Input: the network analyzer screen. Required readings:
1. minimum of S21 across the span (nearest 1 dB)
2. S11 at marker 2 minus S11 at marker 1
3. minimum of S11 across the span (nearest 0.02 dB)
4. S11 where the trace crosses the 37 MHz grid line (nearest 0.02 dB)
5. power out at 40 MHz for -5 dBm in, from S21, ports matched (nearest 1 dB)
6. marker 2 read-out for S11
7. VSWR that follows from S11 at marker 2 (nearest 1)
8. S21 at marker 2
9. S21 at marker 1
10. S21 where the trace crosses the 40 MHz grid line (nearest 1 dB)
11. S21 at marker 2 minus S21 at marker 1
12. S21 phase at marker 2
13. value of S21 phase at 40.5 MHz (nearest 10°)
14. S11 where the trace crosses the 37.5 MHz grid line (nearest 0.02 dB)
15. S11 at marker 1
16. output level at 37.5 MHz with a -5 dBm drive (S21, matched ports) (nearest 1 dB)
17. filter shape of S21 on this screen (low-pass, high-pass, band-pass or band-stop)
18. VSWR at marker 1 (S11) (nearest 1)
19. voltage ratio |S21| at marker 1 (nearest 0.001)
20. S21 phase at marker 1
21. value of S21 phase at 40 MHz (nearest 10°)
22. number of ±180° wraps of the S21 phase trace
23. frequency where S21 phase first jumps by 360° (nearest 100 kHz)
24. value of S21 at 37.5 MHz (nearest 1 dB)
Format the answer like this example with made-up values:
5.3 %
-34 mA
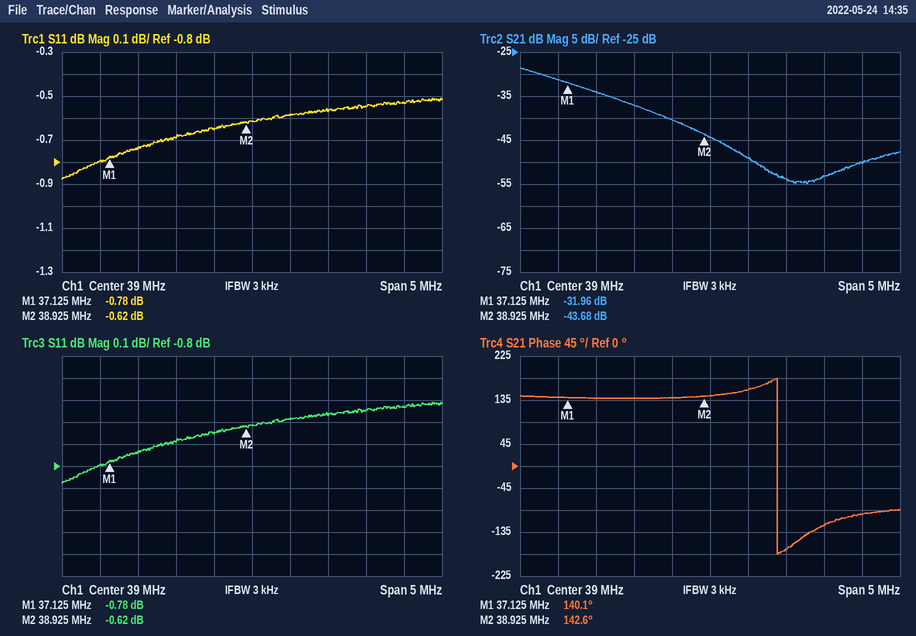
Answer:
-55 dB
0.16 dB
-0.88 dB
-0.80 dB
-59 dBm
-0.62 dB
28
-43.68 dB
-31.96 dB
-54 dB
-11.72 dB
142.6°
-120°
-0.74 dB
-0.78 dB
-39 dBm
low-pass
22
0.025
140.1°
-170°
1
39.9 MHz
-34 dB
